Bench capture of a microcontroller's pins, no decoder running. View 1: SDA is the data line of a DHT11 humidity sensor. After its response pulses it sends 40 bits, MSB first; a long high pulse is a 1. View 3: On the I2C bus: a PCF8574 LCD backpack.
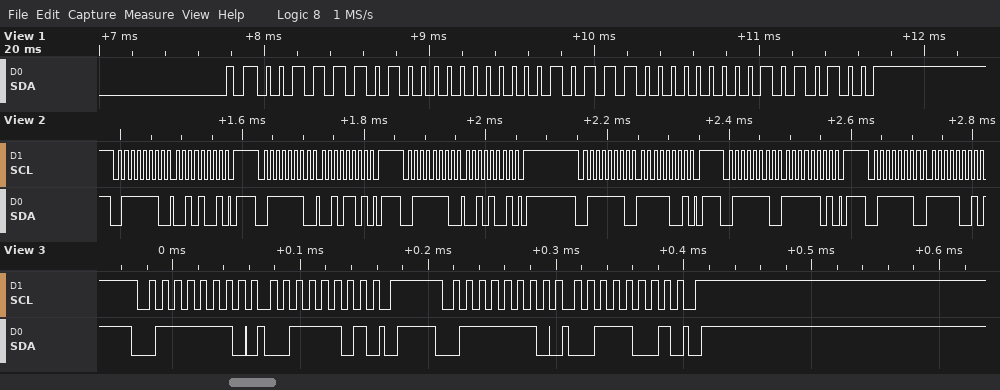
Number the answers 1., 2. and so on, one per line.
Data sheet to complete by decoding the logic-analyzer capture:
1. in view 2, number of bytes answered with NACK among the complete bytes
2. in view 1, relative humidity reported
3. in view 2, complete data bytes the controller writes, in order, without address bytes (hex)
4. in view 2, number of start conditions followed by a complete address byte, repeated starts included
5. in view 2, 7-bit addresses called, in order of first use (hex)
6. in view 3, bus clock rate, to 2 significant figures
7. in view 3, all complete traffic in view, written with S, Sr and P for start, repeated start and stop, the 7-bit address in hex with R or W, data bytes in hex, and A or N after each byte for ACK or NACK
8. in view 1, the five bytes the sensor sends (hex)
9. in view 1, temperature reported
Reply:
1. 0
2. 61 %
3. 29 2D 29 F9 FD F9
4. 6
5. 0x3F
6. 100 kHz
7. S 3FW A 3D A P S 3FW A 39 A P
8. 3D 00 17 00 54
9. 23.0 °C
